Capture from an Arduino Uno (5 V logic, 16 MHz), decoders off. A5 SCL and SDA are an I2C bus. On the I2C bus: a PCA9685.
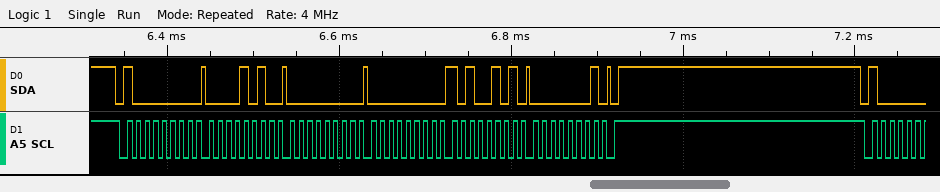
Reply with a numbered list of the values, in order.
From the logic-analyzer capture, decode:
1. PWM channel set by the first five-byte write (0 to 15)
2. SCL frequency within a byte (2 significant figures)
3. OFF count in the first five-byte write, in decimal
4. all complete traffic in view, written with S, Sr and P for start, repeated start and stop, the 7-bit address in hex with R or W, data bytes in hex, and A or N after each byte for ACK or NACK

1. 1
2. 100 kHz
3. 421
4. S 40W A 0A A 00 A 00 A A5 A 01 A P
